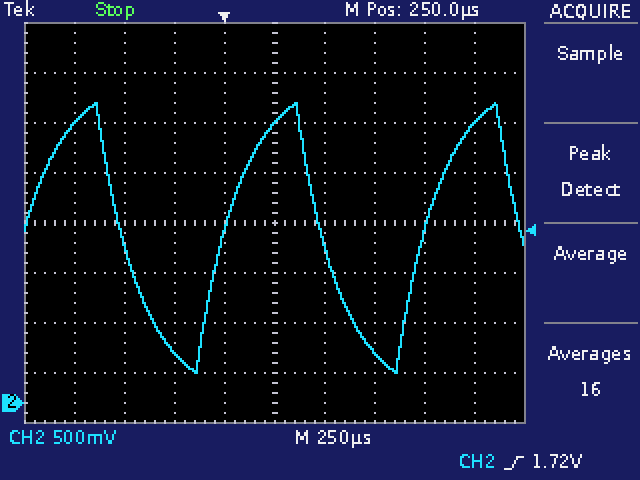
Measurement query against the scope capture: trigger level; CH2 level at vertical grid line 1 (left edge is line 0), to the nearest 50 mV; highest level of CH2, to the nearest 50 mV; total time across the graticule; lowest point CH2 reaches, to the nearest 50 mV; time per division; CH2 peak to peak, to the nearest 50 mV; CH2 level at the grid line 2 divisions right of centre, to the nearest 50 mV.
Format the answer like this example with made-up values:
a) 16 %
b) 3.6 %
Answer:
a) 1.72 V
b) 2.80 V
c) 3.00 V
d) 2.5 ms
e) 300 mV
f) 250 µs
g) 2.70 V
h) 500 mV
